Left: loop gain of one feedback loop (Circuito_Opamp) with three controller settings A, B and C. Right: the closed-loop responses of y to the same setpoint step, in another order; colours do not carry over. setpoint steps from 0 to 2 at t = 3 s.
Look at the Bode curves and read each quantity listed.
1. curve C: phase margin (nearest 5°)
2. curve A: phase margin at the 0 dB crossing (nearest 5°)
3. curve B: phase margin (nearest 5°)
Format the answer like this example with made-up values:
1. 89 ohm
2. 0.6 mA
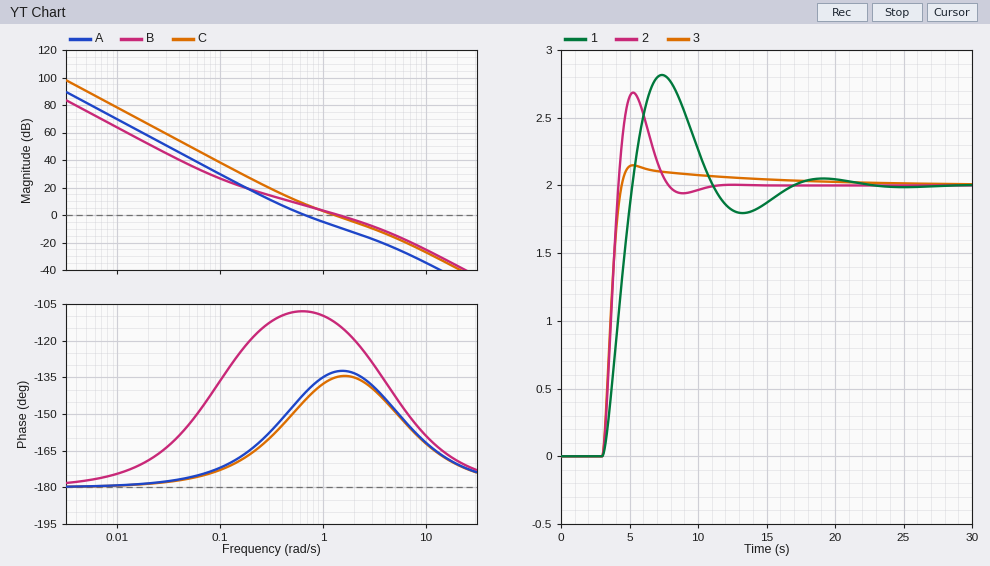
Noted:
1. 45°
2. 40°
3. 65°
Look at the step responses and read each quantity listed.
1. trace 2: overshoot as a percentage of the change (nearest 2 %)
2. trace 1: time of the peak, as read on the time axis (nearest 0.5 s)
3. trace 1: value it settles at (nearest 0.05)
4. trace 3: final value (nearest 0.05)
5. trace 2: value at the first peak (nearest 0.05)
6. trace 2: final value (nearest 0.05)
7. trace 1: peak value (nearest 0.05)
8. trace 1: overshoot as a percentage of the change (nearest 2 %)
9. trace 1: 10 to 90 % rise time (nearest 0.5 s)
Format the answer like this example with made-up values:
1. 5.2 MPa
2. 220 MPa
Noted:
1. 34 %
2. 7.5 s
3. 2.00
4. 2.00
5. 2.70
6. 2.00
7. 2.80
8. 40 %
9. 1.5 s
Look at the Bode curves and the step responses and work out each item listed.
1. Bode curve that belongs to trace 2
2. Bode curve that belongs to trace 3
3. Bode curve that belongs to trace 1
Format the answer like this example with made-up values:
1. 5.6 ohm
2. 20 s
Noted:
1. C
2. B
3. A
